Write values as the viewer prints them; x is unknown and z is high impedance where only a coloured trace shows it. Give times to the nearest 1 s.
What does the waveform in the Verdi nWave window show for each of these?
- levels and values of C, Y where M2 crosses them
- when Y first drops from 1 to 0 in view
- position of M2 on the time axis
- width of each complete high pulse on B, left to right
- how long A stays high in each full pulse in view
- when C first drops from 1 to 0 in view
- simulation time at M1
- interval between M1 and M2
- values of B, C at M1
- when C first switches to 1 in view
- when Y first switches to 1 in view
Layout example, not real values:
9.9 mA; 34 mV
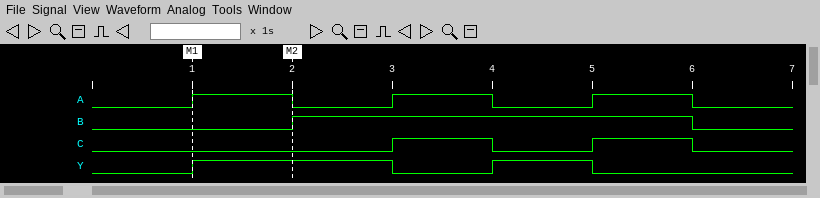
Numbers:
C=0, Y=1; 3 s; 2 s; 4 s; 1 s, 1 s, 1 s; 4 s; 1 s; 1 s; B=0, C=0; 3 s; 1 s
